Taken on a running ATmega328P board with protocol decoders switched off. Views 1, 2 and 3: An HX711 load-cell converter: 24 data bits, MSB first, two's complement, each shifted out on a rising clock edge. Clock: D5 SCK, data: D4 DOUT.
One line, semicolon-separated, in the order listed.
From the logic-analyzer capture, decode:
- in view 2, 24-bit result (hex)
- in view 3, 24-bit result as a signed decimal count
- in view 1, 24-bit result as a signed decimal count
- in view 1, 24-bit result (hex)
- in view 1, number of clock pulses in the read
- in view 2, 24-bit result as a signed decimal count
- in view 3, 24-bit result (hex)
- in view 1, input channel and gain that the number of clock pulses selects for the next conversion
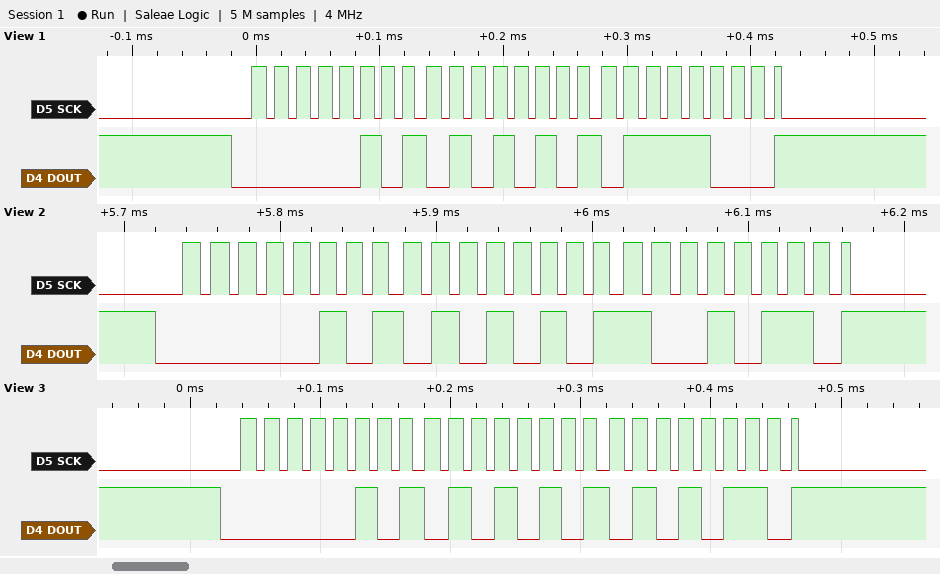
0x055596; 349526; 349560; 0x055578; 25; 349590; 0x055556; channel A, gain 128
